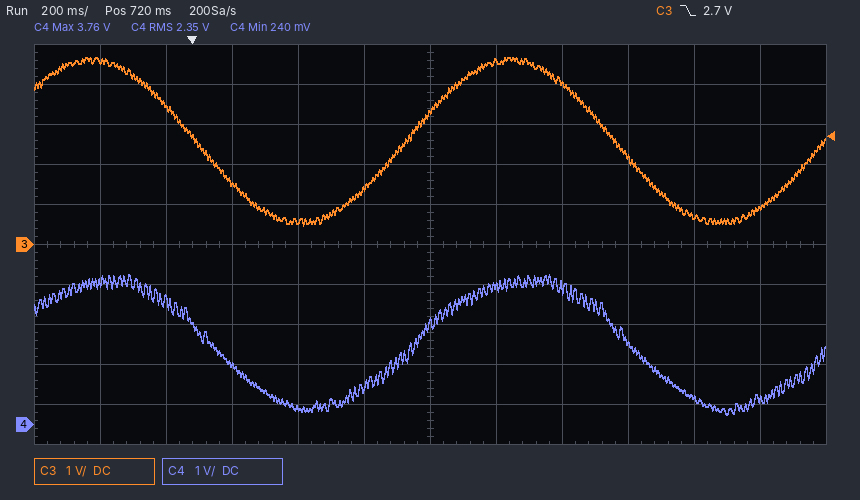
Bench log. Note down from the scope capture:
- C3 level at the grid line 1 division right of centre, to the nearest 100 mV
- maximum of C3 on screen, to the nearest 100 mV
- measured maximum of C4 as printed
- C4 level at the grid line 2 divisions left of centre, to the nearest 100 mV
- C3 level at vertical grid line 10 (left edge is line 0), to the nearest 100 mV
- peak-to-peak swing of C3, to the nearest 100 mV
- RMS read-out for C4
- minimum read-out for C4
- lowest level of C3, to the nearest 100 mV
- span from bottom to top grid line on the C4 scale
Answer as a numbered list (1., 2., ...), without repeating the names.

1. 4.6 V
2. 4.7 V
3. 3.76 V
4. 400 mV
5. 700 mV
6. 4.2 V
7. 2.35 V
8. 240 mV
9. 500 mV
10. 10 V
